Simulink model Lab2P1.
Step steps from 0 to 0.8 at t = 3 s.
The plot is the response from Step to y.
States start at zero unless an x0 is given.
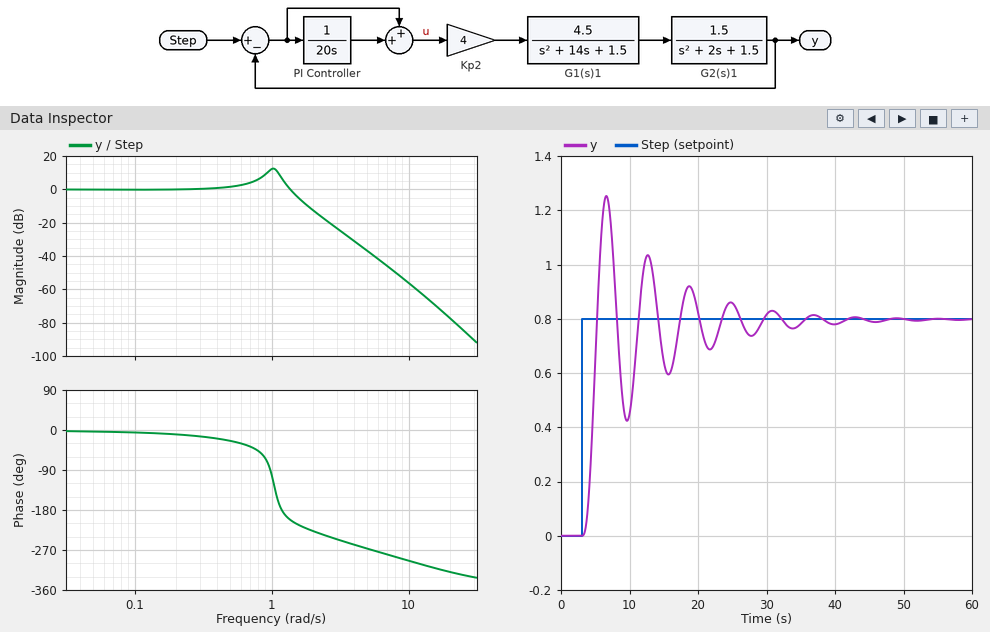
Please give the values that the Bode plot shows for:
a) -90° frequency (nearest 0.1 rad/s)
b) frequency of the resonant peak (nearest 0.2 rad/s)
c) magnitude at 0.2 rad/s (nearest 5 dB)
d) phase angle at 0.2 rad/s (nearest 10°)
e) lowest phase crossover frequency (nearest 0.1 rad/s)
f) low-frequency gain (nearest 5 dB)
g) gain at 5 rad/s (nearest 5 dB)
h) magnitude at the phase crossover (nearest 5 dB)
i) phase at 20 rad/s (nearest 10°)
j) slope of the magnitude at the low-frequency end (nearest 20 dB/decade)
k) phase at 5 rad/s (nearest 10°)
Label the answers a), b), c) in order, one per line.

a) 1.0 rad/s
b) 1.0 rad/s
c) 0 dB
d) -10°
e) 1.2 rad/s
f) 0 dB
g) -35 dB
h) 5 dB
i) -320°
j) 0 dB/decade
k) -270°
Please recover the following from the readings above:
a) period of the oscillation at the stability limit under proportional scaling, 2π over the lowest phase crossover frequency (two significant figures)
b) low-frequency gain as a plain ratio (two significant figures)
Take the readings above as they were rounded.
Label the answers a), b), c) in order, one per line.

a) 5.2 s
b) 1.0
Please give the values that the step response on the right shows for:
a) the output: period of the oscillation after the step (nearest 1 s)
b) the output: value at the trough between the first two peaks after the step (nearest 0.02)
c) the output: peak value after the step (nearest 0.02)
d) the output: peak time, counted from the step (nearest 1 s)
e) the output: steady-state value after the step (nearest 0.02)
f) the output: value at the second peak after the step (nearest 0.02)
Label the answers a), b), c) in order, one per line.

a) 6 s
b) 0.42
c) 1.26
d) 4 s
e) 0.80
f) 1.04
